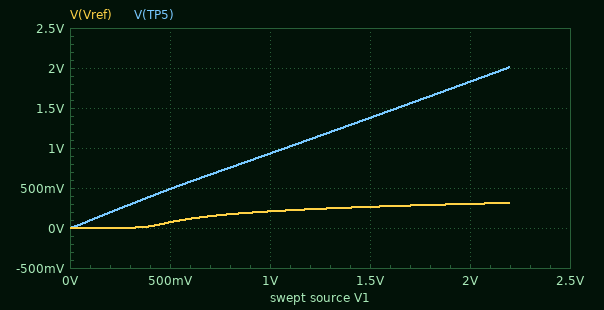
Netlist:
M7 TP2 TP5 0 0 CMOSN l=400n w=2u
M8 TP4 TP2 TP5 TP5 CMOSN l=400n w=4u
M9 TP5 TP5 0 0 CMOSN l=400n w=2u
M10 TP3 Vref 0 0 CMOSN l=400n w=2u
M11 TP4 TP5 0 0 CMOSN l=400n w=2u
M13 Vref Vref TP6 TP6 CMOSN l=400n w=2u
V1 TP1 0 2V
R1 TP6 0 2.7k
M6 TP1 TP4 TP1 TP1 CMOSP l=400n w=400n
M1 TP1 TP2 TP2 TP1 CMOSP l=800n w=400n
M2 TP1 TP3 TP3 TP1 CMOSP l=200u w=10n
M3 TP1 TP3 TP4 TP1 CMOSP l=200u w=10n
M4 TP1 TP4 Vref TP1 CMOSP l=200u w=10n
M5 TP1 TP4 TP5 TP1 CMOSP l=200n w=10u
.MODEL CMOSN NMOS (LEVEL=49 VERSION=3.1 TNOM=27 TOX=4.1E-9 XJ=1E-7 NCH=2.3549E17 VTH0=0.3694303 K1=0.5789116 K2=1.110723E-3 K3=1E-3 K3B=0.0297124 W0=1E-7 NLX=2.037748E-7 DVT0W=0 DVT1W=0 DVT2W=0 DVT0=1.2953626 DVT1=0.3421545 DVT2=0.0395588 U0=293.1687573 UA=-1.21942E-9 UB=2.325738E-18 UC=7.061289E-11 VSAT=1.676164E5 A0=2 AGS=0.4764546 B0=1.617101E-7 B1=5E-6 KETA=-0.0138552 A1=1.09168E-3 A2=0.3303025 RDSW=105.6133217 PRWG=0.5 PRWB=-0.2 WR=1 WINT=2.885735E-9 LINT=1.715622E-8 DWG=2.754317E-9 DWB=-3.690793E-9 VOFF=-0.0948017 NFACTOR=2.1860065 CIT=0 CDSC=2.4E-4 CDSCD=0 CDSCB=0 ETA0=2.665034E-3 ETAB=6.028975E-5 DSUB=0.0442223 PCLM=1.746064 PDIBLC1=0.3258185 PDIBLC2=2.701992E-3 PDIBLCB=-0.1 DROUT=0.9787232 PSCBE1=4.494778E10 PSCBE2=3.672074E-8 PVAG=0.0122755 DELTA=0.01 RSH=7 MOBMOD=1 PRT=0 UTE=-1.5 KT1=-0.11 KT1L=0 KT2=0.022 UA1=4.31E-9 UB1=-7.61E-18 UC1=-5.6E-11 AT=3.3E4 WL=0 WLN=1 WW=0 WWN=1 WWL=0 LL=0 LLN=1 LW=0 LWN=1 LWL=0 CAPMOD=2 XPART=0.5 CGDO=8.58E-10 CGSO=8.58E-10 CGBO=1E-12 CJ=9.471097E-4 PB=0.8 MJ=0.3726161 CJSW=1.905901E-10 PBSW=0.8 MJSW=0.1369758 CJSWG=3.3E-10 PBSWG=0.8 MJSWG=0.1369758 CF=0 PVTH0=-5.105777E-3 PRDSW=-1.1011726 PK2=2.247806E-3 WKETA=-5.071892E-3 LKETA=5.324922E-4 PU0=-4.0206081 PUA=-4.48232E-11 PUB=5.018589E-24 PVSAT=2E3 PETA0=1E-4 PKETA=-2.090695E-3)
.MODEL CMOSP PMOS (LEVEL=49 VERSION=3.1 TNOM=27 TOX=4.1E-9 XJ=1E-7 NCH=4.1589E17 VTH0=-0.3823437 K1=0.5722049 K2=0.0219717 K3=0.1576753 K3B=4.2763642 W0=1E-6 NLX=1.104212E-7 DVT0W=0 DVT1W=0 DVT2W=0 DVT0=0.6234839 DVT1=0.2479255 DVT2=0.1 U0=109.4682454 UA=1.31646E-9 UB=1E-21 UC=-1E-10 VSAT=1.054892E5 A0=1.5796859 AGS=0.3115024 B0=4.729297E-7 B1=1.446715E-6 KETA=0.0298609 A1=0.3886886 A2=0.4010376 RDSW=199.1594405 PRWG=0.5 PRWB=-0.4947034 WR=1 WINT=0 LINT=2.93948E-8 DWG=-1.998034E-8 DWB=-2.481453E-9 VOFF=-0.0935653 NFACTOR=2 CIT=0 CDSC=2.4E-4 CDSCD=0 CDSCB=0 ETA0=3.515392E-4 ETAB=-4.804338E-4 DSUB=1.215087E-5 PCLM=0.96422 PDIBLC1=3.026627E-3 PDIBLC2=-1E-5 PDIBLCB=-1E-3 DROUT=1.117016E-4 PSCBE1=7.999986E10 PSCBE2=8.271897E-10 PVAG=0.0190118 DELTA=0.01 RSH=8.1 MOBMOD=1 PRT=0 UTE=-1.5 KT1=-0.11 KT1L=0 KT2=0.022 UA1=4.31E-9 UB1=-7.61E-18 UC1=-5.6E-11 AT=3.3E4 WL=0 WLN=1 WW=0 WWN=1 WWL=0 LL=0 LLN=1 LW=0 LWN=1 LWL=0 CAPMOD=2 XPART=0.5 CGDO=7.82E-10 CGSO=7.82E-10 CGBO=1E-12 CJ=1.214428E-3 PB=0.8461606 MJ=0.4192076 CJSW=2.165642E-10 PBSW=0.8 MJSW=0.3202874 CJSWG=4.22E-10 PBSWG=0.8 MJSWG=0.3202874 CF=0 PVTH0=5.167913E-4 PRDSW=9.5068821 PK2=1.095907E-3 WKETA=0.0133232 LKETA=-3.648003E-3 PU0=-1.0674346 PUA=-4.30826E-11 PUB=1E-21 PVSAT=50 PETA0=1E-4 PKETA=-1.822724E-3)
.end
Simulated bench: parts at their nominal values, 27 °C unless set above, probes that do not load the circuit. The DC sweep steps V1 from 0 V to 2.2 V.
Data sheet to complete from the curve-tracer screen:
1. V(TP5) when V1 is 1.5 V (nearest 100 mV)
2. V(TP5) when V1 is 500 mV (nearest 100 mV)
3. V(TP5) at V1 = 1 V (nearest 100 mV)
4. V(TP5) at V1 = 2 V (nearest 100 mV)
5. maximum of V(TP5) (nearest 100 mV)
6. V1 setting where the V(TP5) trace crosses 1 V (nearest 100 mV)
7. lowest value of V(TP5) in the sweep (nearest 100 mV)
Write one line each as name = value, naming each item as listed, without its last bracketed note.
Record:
V(TP5) when V1 is 1.5 V = 1.4 V
V(TP5) when V1 is 500 mV = 500 mV
V(TP5) at V1 = 1 V = 900 mV
V(TP5) at V1 = 2 V = 1.8 V
maximum of V(TP5) = 2.0 V
V1 setting where the V(TP5) trace crosses 1 V = 1.1 V
lowest value of V(TP5) in the sweep = 0 V
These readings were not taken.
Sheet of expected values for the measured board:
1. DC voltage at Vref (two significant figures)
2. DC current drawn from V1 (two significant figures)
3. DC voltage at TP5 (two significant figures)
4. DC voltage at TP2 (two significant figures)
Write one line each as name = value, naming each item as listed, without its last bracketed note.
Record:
DC voltage at Vref = 300 mV
DC current drawn from V1 = 710 µA
DC voltage at TP5 = 1.8 V
DC voltage at TP2 = 20 mV
